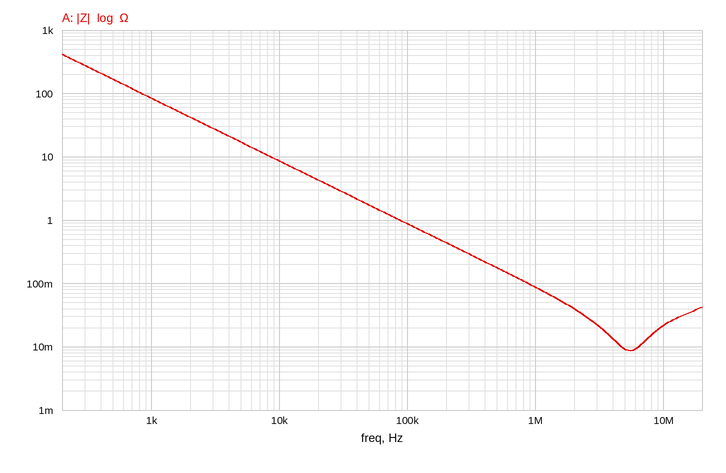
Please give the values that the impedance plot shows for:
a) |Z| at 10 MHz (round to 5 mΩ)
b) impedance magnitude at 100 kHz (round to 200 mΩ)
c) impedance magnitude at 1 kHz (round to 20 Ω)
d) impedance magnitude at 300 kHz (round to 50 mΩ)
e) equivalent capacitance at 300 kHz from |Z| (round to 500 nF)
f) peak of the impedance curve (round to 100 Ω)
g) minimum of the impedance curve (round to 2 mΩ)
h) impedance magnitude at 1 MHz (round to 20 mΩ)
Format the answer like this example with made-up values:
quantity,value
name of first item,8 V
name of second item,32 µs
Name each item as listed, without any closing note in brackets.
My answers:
quantity,value
|Z| at 10 MHz,20 mΩ
impedance magnitude at 100 kHz,800 mΩ
impedance magnitude at 1 kHz,80 Ω
impedance magnitude at 300 kHz,300 mΩ
equivalent capacitance at 300 kHz from |Z|,2.0 µF
peak of the impedance curve,400 Ω
minimum of the impedance curve,8 mΩ
impedance magnitude at 1 MHz,80 mΩ
